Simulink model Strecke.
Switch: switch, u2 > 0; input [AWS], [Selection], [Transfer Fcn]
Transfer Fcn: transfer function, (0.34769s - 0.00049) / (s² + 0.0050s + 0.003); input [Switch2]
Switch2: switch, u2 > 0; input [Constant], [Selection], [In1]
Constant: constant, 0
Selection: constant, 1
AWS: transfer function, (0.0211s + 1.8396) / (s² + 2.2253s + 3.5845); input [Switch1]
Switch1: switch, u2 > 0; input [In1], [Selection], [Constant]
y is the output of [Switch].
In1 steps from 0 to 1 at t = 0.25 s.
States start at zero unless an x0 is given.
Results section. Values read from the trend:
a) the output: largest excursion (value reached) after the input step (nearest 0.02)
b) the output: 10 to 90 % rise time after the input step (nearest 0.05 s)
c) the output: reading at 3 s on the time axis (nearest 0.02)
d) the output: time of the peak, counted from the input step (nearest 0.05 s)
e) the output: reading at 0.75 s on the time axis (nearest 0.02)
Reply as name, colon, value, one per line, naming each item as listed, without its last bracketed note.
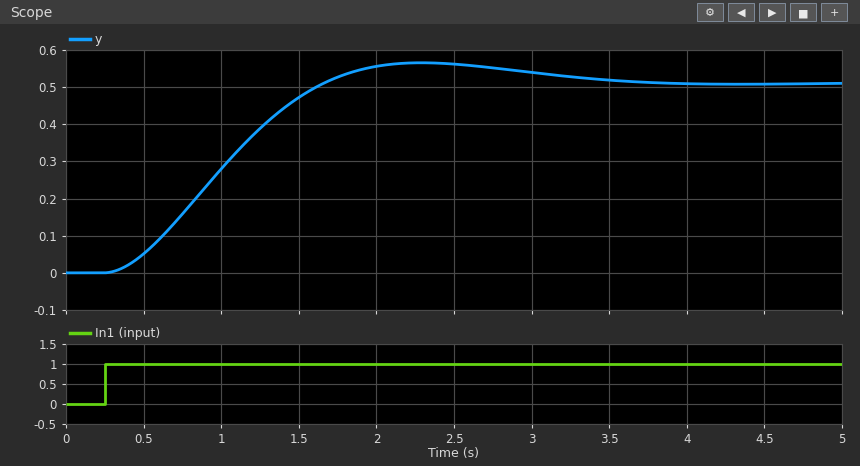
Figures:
the output: largest excursion (value reached) after the input step: 0.56
the output: 10 to 90 % rise time after the input step: 0.95 s
the output: reading at 3 s on the time axis: 0.54
the output: time of the peak, counted from the input step: 2.05 s
the output: reading at 0.75 s on the time axis: 0.16
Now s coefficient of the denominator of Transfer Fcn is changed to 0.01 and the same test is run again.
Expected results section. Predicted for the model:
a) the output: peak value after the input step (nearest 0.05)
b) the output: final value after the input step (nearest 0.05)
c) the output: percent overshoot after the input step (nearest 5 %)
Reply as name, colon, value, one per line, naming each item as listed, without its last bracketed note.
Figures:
the output: peak value after the input step: 0.55
the output: final value after the input step: 0.50
the output: percent overshoot after the input step: 10 %
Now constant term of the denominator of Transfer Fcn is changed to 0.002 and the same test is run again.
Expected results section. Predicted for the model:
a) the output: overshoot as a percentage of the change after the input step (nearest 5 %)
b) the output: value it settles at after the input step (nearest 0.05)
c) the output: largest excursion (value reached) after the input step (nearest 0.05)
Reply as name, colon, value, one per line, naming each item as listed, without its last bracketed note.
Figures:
the output: overshoot as a percentage of the change after the input step: 10 %
the output: value it settles at after the input step: 0.50
the output: largest excursion (value reached) after the input step: 0.55
